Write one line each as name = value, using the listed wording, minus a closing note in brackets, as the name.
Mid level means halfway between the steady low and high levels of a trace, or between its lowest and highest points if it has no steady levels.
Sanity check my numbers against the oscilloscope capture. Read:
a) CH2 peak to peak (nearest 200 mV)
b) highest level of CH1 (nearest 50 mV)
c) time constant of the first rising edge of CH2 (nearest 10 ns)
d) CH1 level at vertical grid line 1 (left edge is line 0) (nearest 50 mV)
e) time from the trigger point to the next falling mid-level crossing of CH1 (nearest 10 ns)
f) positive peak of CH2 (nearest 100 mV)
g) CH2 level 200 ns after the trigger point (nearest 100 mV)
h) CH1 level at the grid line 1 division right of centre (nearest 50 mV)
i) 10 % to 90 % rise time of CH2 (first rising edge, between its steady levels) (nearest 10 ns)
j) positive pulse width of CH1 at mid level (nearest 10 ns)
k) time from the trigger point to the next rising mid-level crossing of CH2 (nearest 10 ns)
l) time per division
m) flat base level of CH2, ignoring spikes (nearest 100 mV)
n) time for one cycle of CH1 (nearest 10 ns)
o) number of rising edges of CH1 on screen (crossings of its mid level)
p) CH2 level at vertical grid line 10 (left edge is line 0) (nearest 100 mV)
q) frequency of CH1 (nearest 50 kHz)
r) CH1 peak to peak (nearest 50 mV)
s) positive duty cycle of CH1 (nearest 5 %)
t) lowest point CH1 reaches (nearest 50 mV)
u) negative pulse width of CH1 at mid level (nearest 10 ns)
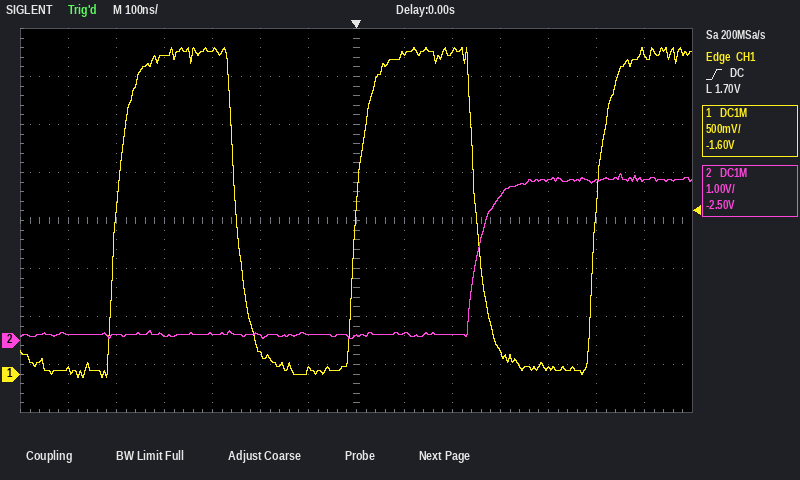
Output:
CH2 peak to peak = 3.4 V
highest level of CH1 = 3.40 V
time constant of the first rising edge of CH2 = 30 ns
CH1 level at vertical grid line 1 (left edge is line 0) = 50 mV
time from the trigger point to the next falling mid-level crossing of CH1 = 250 ns
positive peak of CH2 = 3.5 V
CH2 level 200 ns after the trigger point = 100 mV
CH1 level at the grid line 1 division right of centre = 3.35 V
10 % to 90 % rise time of CH2 (first rising edge, between its steady levels) = 70 ns
positive pulse width of CH1 at mid level = 250 ns
time from the trigger point to the next rising mid-level crossing of CH2 = 250 ns
time per division = 100 ns
flat base level of CH2, ignoring spikes = 100 mV
time for one cycle of CH1 = 500 ns
number of rising edges of CH1 on screen = 3
CH2 level at vertical grid line 10 (left edge is line 0) = 3.0 V
frequency of CH1 = 2.00 MHz
CH1 peak to peak = 3.45 V
positive duty cycle of CH1 = 50 %
lowest point CH1 reaches = -50 mV
negative pulse width of CH1 at mid level = 250 ns
